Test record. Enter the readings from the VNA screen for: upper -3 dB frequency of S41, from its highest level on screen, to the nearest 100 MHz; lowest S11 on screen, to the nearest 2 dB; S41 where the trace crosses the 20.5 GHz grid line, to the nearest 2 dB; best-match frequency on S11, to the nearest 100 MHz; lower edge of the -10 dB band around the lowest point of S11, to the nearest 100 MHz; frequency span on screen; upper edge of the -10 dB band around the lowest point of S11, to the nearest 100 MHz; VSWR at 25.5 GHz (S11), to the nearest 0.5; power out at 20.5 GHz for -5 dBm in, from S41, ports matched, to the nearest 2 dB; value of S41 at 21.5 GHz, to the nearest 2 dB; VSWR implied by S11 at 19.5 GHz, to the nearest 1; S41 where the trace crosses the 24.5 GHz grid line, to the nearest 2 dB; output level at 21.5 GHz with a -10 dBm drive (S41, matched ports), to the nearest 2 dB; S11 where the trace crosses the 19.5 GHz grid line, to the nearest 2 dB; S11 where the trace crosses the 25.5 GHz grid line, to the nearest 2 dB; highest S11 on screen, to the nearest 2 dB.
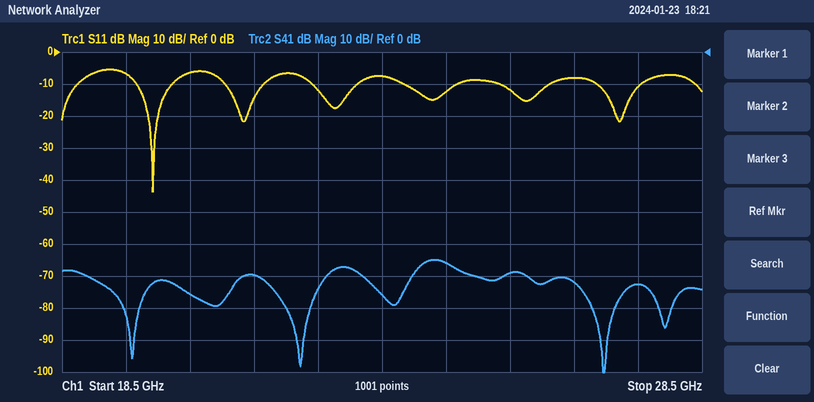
24.7 GHz
-44 dB
-76 dB
19.9 GHz
19.7 GHz
10 GHz
20.2 GHz
1.5
-80 dBm
-70 dB
3
-66 dB
-80 dBm
-6 dB
-12 dB
-6 dB
